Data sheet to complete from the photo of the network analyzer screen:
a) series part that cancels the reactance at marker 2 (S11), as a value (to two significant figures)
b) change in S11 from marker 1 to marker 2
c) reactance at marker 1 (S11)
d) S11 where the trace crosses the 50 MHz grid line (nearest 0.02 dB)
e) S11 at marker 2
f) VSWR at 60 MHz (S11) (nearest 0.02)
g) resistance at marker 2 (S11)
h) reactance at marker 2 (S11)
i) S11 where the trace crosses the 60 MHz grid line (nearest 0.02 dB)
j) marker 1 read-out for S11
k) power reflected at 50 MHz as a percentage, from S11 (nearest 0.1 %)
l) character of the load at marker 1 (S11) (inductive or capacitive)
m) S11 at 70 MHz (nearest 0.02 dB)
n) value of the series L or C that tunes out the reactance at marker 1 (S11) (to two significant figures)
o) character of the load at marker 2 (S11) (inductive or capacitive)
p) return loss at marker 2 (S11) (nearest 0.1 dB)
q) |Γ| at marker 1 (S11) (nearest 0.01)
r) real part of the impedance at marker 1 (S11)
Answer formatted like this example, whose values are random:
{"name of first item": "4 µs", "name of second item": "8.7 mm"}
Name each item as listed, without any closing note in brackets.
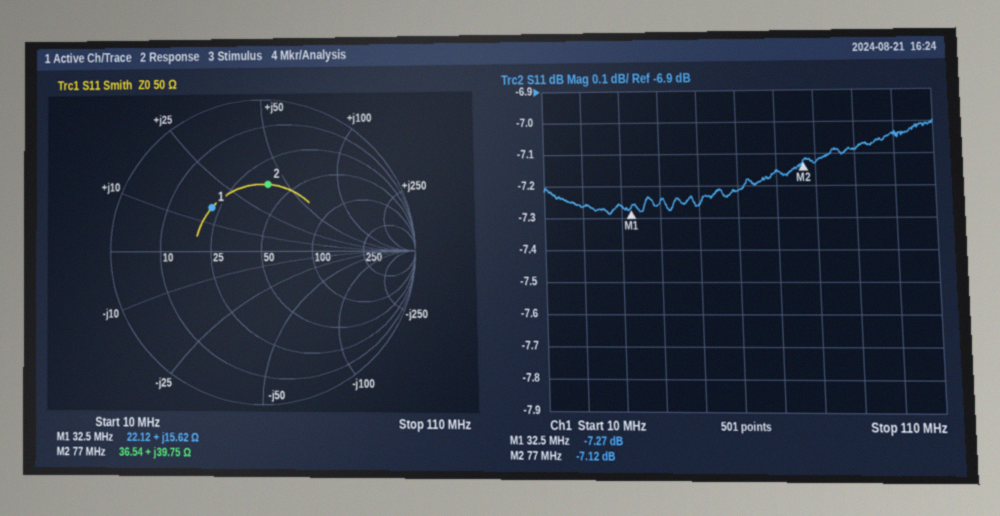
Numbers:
{"series part that cancels the reactance at marker 2 (S11), as a value": "52 pF", "change in S11 from marker 1 to marker 2": "0.15 dB", "reactance at marker 1": "+15.62 Ω", "S11 where the trace crosses the 50 MHz grid line": "-7.26 dB", "S11 at marker 2": "-7.12 dB", "VSWR at 60 MHz (S11)": "2.54", "resistance at marker 2": "36.54 Ω", "reactance at marker 2": "+39.75 Ω", "S11 where the trace crosses the 60 MHz grid line": "-7.22 dB", "marker 1 read-out for S11": "-7.27 dB", "power reflected at 50 MHz as a percentage, from S11": "18.8 %", "character of the load at marker 1 (S11)": "inductive", "S11 at 70 MHz": "-7.16 dB", "value of the series L or C that tunes out the reactance at marker 1 (S11)": "310 pF", "character of the load at marker 2 (S11)": "inductive", "return loss at marker 2 (S11)": "7.1 dB", "|Γ| at marker 1 (S11)": "0.43", "real part of the impedance at marker 1": "22.12 Ω"}
